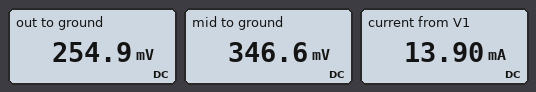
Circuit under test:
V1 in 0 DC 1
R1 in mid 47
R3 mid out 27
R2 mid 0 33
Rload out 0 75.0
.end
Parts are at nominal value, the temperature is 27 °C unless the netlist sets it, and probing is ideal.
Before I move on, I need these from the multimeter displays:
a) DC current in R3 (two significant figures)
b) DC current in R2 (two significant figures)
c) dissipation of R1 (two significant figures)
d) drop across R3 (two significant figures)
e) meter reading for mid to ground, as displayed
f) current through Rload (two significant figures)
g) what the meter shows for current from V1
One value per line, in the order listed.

3.4 mA
11 mA
9.1 mW
92 mV
346.6 mV
3.4 mA
13.90 mA
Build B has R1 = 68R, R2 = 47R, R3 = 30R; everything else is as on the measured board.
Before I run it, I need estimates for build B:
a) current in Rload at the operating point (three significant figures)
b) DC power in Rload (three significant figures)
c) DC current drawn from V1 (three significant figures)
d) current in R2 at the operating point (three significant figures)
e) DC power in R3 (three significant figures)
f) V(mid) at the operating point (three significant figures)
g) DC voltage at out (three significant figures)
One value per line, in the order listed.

3.08 mA
710 µW
9.95 mA
6.88 mA
284 µW
323 mV
231 mV
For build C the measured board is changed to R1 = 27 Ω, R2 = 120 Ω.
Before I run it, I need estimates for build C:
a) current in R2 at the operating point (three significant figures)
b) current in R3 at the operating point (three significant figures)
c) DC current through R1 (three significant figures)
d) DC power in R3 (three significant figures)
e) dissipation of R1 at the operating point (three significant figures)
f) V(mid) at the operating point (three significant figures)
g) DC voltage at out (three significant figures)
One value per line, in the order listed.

5.59 mA
6.58 mA
12.2 mA
1.17 mW
4.00 mW
671 mV
494 mV
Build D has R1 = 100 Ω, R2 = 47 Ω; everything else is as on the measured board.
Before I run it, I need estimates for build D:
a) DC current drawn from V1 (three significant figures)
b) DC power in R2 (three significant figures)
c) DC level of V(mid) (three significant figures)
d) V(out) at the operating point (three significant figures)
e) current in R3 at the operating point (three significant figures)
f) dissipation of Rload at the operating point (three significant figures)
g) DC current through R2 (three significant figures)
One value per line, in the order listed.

7.57 mA
1.26 mW
243 mV
179 mV
2.39 mA
427 µW
5.18 mA
